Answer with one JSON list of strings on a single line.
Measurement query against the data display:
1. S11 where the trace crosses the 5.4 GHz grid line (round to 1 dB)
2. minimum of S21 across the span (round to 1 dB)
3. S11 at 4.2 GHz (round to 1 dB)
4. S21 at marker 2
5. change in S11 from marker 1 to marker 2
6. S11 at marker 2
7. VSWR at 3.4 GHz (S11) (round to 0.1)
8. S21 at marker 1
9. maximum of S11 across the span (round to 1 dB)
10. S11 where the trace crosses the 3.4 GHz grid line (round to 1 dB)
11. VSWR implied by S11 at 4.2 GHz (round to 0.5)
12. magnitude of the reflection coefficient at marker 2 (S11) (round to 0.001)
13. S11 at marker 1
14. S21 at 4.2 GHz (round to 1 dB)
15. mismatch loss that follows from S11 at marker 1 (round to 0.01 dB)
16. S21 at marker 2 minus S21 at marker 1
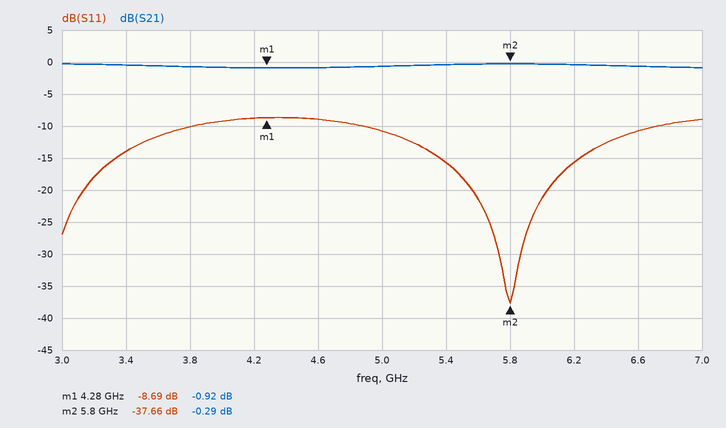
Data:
["-16 dB", "-1 dB", "-9 dB", "-0.29 dB", "-28.97 dB", "-37.66 dB", "1.5", "-0.92 dB", "-9 dB", "-14 dB", "2.0", "0.013", "-8.69 dB", "-1 dB", "0.63 dB", "0.63 dB"]
